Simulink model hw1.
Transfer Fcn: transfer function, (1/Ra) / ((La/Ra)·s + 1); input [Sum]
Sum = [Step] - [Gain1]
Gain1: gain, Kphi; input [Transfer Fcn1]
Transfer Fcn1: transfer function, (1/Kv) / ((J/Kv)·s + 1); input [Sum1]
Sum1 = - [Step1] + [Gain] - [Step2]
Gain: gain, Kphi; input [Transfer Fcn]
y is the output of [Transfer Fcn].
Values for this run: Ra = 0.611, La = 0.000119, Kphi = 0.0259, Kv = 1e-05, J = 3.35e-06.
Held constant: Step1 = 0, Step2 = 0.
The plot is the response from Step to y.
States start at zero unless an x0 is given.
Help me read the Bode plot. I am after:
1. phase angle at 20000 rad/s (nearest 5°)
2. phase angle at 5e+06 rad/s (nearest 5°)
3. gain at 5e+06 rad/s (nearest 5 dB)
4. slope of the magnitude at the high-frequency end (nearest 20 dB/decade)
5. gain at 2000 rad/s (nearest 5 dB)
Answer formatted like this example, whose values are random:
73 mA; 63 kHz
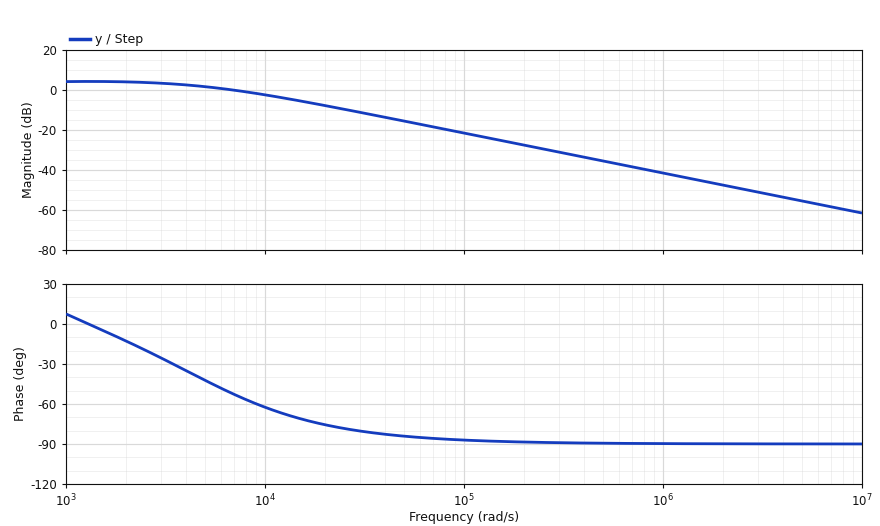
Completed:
-75°; -90°; -55 dB; -20 dB/decade; 5 dB
